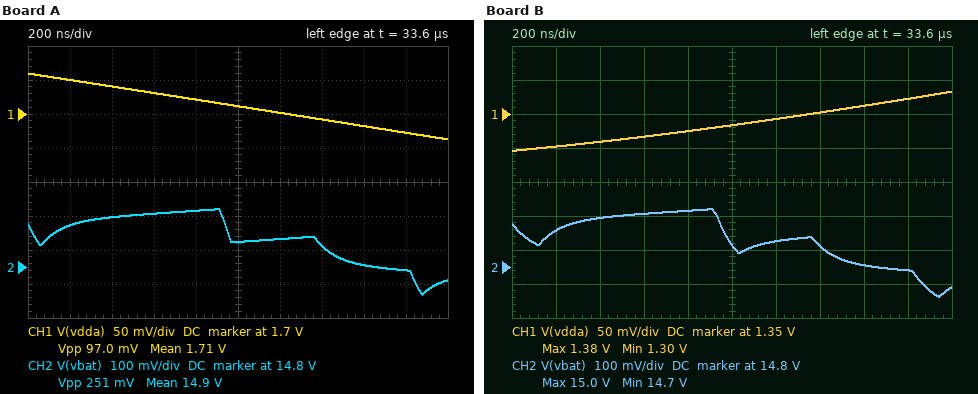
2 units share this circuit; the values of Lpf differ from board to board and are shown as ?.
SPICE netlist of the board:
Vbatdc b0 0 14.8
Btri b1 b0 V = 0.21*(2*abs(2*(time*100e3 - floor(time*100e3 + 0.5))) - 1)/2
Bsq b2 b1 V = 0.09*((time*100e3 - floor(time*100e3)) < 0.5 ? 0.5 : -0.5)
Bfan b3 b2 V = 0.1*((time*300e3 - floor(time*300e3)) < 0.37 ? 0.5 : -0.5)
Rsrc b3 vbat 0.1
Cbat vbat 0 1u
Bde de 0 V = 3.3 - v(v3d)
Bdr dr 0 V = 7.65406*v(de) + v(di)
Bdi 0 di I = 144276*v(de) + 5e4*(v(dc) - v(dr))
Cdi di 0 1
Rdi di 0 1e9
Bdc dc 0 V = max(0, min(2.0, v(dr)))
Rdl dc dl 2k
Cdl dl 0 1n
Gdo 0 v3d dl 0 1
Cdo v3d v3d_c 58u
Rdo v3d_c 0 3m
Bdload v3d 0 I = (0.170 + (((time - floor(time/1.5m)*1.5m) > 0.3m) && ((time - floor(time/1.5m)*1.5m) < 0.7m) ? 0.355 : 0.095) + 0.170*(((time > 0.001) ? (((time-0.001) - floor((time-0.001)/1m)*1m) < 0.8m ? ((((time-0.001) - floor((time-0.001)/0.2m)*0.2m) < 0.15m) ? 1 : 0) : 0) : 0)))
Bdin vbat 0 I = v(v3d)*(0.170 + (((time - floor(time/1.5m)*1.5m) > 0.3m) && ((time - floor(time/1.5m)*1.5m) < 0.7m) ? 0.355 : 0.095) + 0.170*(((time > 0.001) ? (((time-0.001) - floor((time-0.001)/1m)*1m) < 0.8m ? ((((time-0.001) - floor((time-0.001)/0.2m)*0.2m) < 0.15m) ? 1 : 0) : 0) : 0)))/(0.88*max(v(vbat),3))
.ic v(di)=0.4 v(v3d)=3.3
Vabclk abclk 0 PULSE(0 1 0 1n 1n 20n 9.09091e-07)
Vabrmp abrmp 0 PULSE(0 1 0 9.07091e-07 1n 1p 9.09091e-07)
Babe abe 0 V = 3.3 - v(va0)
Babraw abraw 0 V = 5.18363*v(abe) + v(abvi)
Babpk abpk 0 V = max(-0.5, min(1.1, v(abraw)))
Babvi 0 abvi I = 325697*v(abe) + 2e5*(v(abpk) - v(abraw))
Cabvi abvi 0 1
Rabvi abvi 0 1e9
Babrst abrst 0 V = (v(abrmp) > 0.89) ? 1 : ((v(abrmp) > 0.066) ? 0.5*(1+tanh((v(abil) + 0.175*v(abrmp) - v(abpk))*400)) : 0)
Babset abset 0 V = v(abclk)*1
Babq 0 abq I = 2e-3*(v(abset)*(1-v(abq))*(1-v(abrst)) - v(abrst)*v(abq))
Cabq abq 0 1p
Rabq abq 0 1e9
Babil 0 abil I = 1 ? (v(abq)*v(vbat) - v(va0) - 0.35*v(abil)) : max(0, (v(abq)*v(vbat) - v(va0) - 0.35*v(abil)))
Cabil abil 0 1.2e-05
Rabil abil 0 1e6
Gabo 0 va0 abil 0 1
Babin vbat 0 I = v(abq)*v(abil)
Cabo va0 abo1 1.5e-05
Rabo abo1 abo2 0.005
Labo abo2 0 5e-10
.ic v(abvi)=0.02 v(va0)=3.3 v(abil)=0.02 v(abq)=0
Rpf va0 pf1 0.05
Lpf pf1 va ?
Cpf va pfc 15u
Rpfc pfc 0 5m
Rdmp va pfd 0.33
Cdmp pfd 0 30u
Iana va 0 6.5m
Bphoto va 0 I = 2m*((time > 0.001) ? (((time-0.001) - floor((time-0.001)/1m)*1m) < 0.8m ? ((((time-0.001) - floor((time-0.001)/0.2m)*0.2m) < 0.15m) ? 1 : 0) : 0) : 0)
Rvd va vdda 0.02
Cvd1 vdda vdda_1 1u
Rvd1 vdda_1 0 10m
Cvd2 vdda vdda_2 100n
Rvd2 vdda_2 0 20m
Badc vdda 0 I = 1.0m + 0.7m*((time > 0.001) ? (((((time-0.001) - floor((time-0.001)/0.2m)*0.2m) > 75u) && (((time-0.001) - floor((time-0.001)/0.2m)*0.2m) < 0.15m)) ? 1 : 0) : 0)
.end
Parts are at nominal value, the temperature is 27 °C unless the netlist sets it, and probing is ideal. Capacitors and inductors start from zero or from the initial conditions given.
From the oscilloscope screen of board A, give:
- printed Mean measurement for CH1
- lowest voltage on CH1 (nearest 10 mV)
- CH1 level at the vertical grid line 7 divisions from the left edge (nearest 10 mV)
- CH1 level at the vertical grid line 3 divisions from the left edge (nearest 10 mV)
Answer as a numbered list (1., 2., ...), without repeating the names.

1. 1.71 V
2. 1.66 V
3. 1.69 V
4. 1.73 V
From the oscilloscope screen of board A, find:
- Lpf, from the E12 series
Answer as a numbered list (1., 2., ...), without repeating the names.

1. 6.8 µH
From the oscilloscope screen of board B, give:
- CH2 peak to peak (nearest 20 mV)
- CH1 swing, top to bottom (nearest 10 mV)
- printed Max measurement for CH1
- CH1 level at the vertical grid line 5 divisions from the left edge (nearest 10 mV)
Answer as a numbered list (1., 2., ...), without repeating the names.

1. 260 mV
2. 90 mV
3. 1.38 V
4. 1.33 V
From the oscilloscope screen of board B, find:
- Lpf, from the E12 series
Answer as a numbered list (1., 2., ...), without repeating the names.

1. 820 nH
